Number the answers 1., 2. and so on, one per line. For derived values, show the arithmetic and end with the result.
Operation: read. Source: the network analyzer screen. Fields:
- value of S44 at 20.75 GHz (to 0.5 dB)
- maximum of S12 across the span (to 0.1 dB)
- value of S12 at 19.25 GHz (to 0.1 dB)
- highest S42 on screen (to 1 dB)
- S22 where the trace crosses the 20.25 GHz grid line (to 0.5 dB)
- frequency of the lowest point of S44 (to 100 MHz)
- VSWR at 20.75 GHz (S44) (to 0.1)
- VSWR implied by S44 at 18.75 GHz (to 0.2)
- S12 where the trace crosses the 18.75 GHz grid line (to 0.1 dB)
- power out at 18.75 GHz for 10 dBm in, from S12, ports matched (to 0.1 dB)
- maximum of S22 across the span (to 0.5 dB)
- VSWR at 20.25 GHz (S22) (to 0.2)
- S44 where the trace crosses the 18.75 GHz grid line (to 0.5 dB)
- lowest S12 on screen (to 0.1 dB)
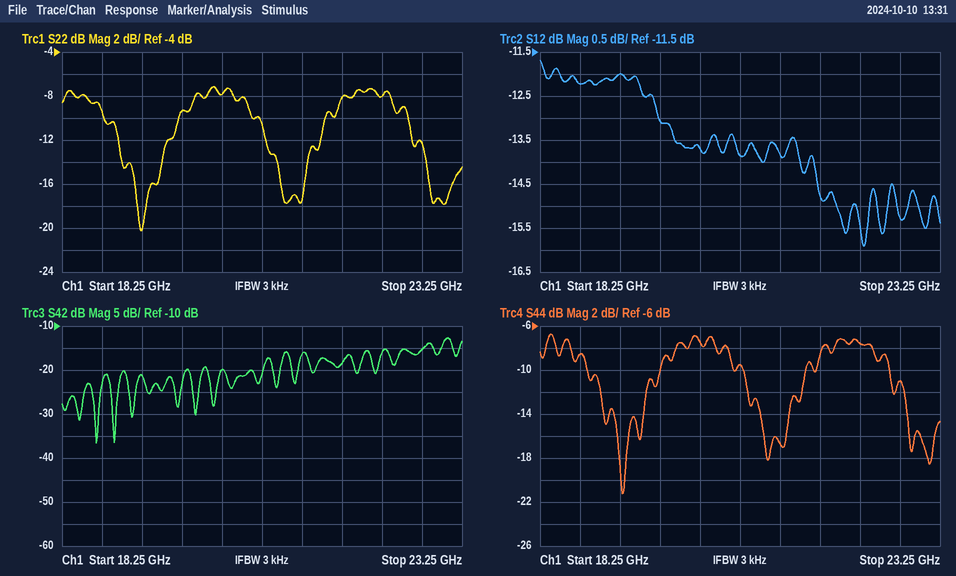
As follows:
1. -9.5 dB
2. -11.7 dB
3. -12.0 dB
4. -13 dB
5. -8.0 dB
6. 19.3 GHz
7. |Γ| = 10^(-9.5/20) = 0.3350; VSWR = (1 + 0.3350)/(1 − 0.3350) ≈ 2.0
8. |Γ| = 10^(-8.5/20) = 0.3758; VSWR = (1 + 0.3758)/(1 − 0.3758) ≈ 2.2
9. -12.2 dB
10. 10 dBm + (-12.2 dB) = -2.2 dBm
11. -7.0 dB
12. |Γ| = 10^(-8/20) = 0.3981; VSWR = (1 + 0.3981)/(1 − 0.3981) ≈ 2.32, so 2.4 to the nearest 0.2
13. -8.5 dB
14. -15.9 dB
